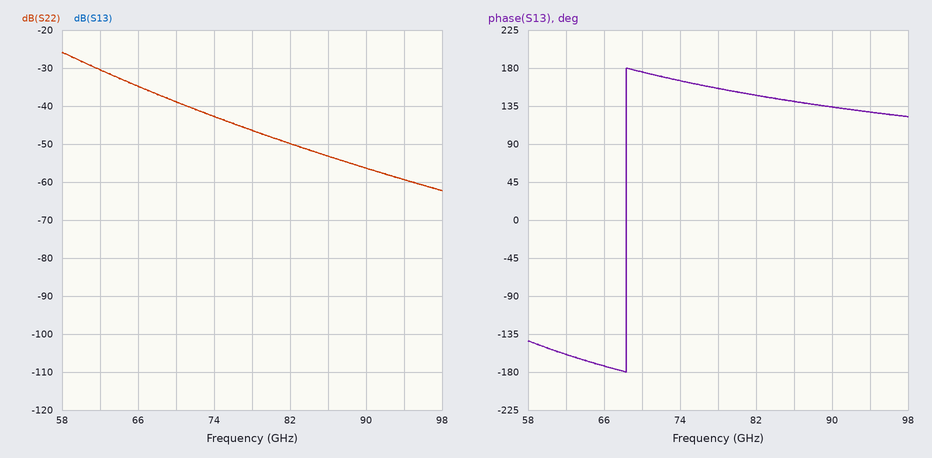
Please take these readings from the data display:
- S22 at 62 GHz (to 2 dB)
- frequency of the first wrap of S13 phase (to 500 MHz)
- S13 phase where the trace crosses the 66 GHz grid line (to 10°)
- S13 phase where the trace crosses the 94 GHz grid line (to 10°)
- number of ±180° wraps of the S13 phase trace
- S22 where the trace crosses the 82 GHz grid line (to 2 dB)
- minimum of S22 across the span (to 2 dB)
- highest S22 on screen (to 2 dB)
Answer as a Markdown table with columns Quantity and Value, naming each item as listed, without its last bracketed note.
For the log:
| Quantity | Value |
|---|---|
| S22 at 62 GHz | -30 dB |
| frequency of the first wrap of S13 phase | 68.5 GHz |
| S13 phase where the trace crosses the 66 GHz grid line | -170° |
| S13 phase where the trace crosses the 94 GHz grid line | 130° |
| number of ±180° wraps of the S13 phase trace | 1 |
| S22 where the trace crosses the 82 GHz grid line | -50 dB |
| minimum of S22 across the span | -62 dB |
| highest S22 on screen | -26 dB |
